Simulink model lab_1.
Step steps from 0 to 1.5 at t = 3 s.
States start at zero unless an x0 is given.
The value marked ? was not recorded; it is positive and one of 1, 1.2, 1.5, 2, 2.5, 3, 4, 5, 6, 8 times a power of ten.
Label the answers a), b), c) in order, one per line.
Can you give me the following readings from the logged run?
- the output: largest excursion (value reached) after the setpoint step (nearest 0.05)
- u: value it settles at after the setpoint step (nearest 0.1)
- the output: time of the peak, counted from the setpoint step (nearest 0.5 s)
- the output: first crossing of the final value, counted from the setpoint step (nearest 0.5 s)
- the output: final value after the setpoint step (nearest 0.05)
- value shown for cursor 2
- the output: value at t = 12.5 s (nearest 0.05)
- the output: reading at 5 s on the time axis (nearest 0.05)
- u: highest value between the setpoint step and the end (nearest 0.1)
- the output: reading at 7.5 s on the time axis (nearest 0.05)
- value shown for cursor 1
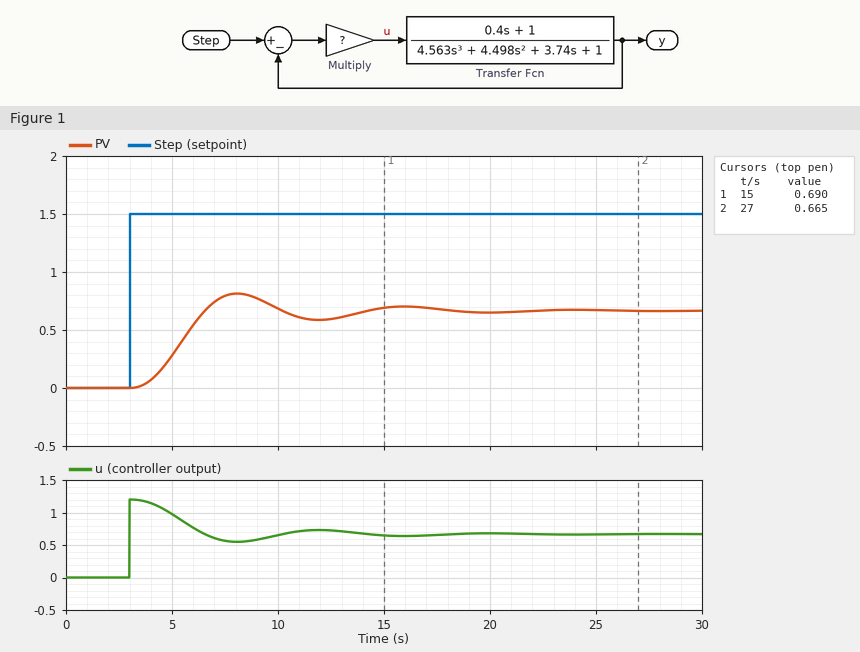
a) 0.80
b) 0.7
c) 5.0 s
d) 3.5 s
e) 0.65
f) 0.665
g) 0.60
h) 0.30
i) 1.2
j) 0.80
k) 0.690
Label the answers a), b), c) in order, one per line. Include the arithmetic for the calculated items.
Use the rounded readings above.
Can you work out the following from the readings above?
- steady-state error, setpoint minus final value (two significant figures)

a) 1.5 - 0.65 = 0.85
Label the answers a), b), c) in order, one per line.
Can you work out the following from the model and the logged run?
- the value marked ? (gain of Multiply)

a) 0.8
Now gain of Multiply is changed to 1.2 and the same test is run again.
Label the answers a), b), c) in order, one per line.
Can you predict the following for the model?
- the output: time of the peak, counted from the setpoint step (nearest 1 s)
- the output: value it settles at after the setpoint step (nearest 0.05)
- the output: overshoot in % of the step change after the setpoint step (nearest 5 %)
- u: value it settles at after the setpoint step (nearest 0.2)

a) 5 s
b) 0.80
c) 30 %
d) 0.8
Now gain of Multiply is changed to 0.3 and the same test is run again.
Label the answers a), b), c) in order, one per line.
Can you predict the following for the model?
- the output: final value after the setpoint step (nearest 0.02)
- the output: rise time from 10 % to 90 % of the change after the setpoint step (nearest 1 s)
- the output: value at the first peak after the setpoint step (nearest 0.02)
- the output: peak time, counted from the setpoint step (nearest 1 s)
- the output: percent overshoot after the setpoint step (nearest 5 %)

a) 0.34
b) 3 s
c) 0.38
d) 6 s
e) 10 %
